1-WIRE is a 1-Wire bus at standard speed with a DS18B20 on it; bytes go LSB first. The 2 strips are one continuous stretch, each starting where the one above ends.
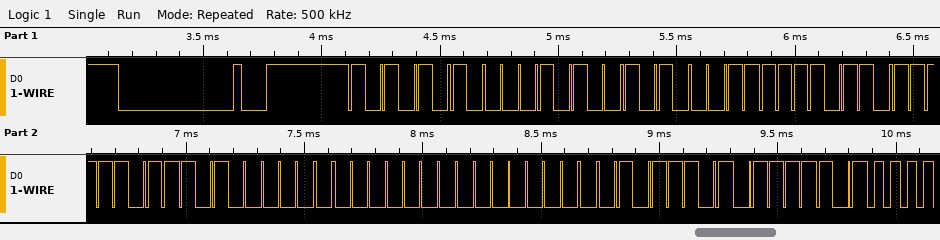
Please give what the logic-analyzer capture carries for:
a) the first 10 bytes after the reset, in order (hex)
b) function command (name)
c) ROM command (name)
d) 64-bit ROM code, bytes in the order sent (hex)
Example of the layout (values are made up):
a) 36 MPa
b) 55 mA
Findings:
a) 55 28 C5 6F DF 05 00 00 BA BE
b) Read Scratchpad
c) Match ROM
d) 28 C5 6F DF 05 00 00 BA
